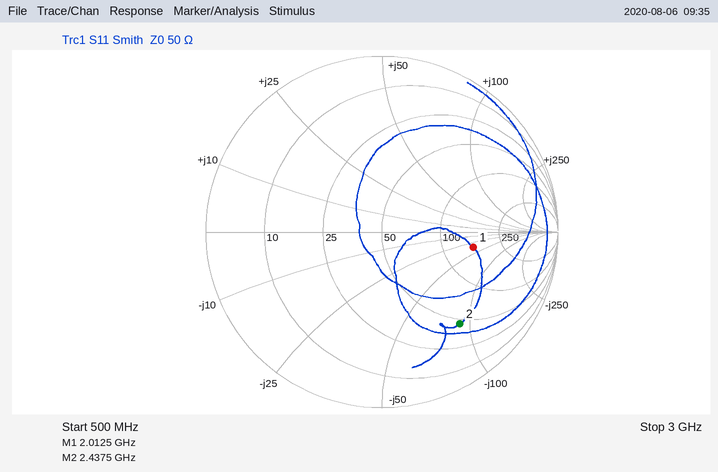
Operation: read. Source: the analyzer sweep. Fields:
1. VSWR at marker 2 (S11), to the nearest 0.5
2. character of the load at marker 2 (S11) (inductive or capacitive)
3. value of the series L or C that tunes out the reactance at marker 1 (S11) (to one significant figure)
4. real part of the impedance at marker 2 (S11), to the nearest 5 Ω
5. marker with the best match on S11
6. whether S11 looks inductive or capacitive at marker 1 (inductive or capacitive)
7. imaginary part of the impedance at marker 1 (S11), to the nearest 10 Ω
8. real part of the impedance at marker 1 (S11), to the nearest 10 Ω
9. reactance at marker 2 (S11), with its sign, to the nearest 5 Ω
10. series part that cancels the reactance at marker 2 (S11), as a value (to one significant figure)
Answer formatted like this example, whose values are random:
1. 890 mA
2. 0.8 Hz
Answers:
1. 5.5
2. capacitive
3. 3 nH
4. 45 Ω
5. marker 1
6. capacitive
7. -40 Ω
8. 150 Ω
9. -90 Ω
10. 6 nH
